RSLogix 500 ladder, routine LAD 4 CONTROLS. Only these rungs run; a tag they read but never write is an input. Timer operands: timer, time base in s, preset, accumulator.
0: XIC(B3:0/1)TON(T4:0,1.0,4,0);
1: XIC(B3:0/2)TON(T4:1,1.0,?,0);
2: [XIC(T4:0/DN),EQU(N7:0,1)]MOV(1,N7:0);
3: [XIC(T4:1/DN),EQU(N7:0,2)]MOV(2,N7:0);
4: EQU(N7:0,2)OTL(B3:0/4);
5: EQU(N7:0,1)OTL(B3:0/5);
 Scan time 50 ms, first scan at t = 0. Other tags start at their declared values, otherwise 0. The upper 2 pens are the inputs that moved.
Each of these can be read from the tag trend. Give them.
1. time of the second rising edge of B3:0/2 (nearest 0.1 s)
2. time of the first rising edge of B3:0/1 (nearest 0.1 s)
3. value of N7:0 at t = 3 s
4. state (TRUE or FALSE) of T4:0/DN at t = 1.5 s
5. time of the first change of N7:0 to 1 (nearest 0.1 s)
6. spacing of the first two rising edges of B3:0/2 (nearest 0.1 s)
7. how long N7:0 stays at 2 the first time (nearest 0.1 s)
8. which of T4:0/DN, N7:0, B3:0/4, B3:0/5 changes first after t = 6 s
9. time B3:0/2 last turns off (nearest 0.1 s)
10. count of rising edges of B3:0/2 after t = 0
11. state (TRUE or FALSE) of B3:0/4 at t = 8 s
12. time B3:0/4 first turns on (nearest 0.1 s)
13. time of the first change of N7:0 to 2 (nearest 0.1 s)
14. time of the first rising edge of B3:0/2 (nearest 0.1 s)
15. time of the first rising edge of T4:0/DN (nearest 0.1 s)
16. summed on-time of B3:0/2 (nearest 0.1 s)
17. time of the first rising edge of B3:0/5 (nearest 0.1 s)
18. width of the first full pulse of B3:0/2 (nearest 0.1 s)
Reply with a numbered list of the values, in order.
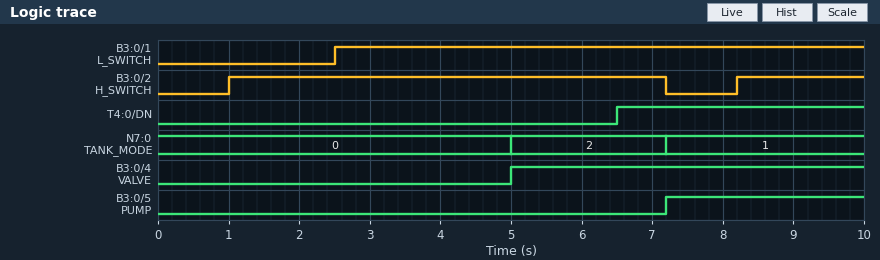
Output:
1. 8.2 s
2. 2.5 s
3. 0
4. FALSE
5. 7.2 s
6. 7.2 s
7. 2.2 s
8. T4:0/DN
9. 7.2 s
10. 2
11. TRUE
12. 5.0 s
13. 5.0 s
14. 1.0 s
15. 6.5 s
16. 8.0 s
17. 7.2 s
18. 6.2 s
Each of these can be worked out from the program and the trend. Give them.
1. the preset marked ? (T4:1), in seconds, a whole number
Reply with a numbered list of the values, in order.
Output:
1. 4 s
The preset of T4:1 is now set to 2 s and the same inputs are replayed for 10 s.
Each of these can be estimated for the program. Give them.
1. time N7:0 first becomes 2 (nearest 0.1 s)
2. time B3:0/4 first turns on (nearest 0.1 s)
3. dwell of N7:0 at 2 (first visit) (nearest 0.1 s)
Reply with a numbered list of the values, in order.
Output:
1. 3.0 s
2. 3.0 s
3. 4.2 s
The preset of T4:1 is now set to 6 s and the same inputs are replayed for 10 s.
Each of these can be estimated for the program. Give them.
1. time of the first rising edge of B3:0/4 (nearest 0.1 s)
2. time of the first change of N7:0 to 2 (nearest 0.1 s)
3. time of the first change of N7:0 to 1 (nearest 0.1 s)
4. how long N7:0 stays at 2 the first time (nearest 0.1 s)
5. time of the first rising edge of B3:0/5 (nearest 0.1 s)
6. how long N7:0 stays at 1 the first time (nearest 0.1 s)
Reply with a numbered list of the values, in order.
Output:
1. 7.0 s
2. 7.0 s
3. 6.5 s
4. 0.2 s
5. 6.5 s
6. 0.5 s
